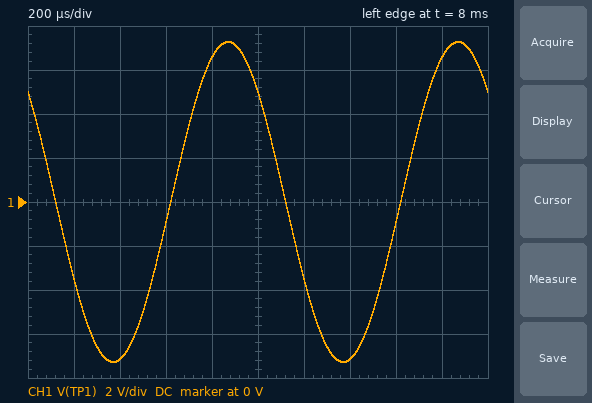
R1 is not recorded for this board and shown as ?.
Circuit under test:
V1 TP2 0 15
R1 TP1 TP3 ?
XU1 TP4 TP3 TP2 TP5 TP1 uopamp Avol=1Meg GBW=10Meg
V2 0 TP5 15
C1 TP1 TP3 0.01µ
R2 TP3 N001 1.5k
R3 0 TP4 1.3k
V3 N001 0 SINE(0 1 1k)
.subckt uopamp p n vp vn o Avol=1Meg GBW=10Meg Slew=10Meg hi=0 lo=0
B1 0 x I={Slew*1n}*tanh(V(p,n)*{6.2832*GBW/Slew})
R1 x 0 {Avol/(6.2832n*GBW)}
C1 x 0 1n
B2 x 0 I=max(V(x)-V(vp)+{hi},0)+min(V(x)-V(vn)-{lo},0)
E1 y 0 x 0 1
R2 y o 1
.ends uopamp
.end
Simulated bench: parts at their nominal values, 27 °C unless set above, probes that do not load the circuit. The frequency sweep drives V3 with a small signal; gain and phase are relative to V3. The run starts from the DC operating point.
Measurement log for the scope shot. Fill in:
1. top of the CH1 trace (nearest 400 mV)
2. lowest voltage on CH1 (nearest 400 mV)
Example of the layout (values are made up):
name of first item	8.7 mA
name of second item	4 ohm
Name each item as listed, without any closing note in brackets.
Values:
top of the CH1 trace	7.2 V
lowest voltage on CH1	-7.2 V
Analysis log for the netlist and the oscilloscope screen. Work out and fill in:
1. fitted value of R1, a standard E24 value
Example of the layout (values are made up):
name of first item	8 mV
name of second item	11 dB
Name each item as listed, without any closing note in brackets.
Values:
fitted value of R1, a standard E24 value	15 kΩ
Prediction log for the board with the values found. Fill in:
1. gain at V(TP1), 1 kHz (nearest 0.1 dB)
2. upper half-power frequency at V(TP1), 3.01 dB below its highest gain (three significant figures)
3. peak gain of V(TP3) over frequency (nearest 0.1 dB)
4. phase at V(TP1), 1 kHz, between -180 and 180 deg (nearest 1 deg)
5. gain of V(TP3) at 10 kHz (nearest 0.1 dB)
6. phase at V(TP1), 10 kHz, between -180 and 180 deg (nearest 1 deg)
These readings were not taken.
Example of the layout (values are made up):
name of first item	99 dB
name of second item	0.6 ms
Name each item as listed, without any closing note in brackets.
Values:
gain at V(TP1), 1 kHz	17.2 dB
upper half-power frequency at V(TP1), 3.01 dB below its highest gain	1.06 kHz
peak gain of V(TP3) over frequency	-59.5 dB
phase at V(TP1), 1 kHz, between -180 and 180 deg	137 deg
gain of V(TP3) at 10 kHz	-59.5 dB
phase at V(TP1), 10 kHz, between -180 and 180 deg	96 deg
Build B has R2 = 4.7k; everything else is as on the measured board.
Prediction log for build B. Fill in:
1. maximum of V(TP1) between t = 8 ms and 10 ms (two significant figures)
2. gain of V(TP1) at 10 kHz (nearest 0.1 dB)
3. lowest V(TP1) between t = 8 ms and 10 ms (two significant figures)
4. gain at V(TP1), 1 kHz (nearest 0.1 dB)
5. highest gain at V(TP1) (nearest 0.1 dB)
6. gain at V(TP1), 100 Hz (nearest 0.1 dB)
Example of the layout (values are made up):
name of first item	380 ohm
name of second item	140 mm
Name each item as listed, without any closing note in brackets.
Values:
maximum of V(TP1) between t = 8 ms and 10 ms	2.3 V
gain of V(TP1) at 10 kHz	-9.5 dB
lowest V(TP1) between t = 8 ms and 10 ms	-2.3 V
gain at V(TP1), 1 kHz	7.3 dB
highest gain at V(TP1)	10.1 dB
gain at V(TP1), 100 Hz	10.0 dB
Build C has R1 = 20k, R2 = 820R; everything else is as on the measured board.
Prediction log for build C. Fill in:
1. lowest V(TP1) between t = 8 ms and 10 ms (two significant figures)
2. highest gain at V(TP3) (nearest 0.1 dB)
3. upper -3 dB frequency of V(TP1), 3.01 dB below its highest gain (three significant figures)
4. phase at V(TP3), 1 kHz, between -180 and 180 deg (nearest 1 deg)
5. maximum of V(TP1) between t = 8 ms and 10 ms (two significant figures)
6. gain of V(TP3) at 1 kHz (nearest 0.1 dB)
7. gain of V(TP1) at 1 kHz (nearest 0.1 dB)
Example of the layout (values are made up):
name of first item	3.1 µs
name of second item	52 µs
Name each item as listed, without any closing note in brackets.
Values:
lowest V(TP1) between t = 8 ms and 10 ms	-15 V
highest gain at V(TP3)	-54.3 dB
upper -3 dB frequency of V(TP1), 3.01 dB below its highest gain	794 Hz
phase at V(TP3), 1 kHz, between -180 and 180 deg	38 deg
maximum of V(TP1) between t = 8 ms and 10 ms	15 V
gain of V(TP3) at 1 kHz	-56.4 dB
gain of V(TP1) at 1 kHz	23.6 dB
